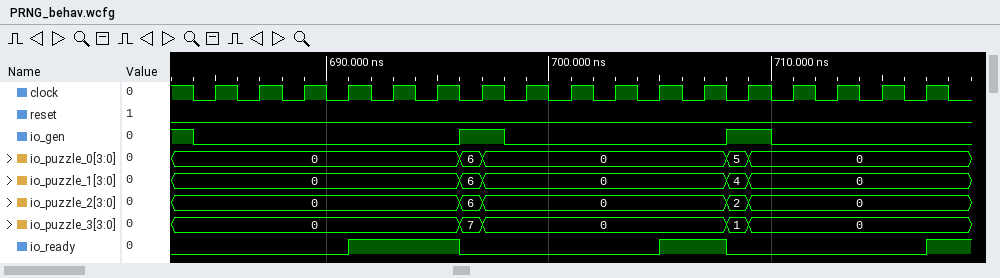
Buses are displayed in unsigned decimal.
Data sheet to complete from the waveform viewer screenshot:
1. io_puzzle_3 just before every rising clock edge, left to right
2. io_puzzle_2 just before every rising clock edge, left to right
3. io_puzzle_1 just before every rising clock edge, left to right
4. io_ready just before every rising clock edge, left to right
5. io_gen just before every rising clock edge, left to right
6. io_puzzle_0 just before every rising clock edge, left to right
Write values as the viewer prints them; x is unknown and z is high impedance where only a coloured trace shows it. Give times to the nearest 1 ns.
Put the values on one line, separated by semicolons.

0, 0, 0, 0, 0, 0, 7, 0, 0, 0, 0, 0, 1, 0, 0, 0, 0; 0, 0, 0, 0, 0, 0, 6, 0, 0, 0, 0, 0, 2, 0, 0, 0, 0; 0, 0, 0, 0, 0, 0, 6, 0, 0, 0, 0, 0, 4, 0, 0, 0, 0; 0 0 0 0 1 1 0 0 0 0 0 1 0 0 0 0 0; 0 0 0 0 0 0 1 0 0 0 0 0 1 0 0 0 0; 0, 0, 0, 0, 0, 0, 6, 0, 0, 0, 0, 0, 5, 0, 0, 0, 0
